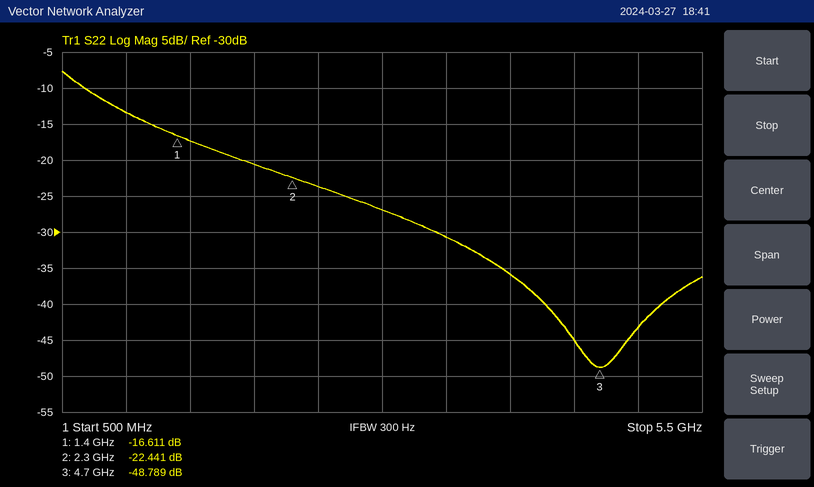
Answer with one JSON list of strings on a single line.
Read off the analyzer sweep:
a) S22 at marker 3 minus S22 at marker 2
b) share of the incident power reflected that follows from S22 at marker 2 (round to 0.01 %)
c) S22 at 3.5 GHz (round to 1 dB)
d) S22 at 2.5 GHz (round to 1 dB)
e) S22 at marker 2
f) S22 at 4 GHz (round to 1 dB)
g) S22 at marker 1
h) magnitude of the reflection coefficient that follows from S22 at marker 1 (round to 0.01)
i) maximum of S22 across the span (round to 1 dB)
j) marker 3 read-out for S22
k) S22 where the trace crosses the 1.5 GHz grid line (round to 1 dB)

["-26.348 dB", "0.57 %", "-31 dB", "-24 dB", "-22.441 dB", "-36 dB", "-16.611 dB", "0.15", "-8 dB", "-48.789 dB", "-17 dB"]
